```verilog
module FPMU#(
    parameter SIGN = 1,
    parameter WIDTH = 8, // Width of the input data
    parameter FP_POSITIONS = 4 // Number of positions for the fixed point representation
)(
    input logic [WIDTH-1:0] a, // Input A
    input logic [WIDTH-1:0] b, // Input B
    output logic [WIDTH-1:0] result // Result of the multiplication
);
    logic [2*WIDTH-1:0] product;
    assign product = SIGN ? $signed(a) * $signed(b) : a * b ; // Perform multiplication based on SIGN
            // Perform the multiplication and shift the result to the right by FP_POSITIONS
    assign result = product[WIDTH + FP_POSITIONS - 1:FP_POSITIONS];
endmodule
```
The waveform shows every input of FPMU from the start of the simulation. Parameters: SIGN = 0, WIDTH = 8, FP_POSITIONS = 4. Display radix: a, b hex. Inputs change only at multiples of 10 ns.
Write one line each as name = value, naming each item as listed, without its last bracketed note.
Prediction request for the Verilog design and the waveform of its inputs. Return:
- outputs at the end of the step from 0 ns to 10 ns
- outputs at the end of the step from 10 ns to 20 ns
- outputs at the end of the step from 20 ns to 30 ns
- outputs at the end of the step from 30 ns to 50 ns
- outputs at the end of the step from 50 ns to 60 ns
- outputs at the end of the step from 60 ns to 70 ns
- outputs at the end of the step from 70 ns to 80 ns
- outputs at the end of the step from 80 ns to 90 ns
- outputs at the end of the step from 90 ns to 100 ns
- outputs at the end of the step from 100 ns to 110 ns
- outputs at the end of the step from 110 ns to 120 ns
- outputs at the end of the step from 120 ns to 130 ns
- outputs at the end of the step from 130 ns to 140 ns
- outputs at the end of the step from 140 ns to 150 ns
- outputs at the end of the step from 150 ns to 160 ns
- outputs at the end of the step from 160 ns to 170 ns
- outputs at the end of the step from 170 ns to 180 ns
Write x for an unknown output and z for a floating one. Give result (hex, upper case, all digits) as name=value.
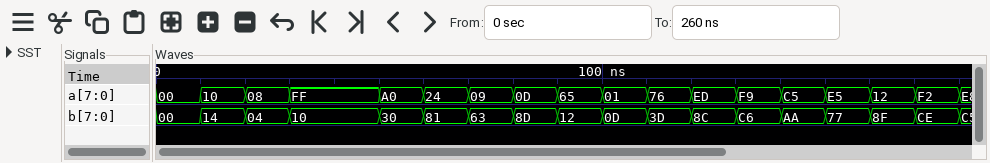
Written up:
outputs at the end of the step from 0 ns to 10 ns = result=00
outputs at the end of the step from 10 ns to 20 ns = result=14
outputs at the end of the step from 20 ns to 30 ns = result=02
outputs at the end of the step from 30 ns to 50 ns = result=FF
outputs at the end of the step from 50 ns to 60 ns = result=E0
outputs at the end of the step from 60 ns to 70 ns = result=22
outputs at the end of the step from 70 ns to 80 ns = result=37
outputs at the end of the step from 80 ns to 90 ns = result=72
outputs at the end of the step from 90 ns to 100 ns = result=71
outputs at the end of the step from 100 ns to 110 ns = result=00
outputs at the end of the step from 110 ns to 120 ns = result=C1
outputs at the end of the step from 120 ns to 130 ns = result=19
outputs at the end of the step from 130 ns to 140 ns = result=09
outputs at the end of the step from 140 ns to 150 ns = result=2D
outputs at the end of the step from 150 ns to 160 ns = result=A7
outputs at the end of the step from 160 ns to 170 ns = result=A0
outputs at the end of the step from 170 ns to 180 ns = result=2B
